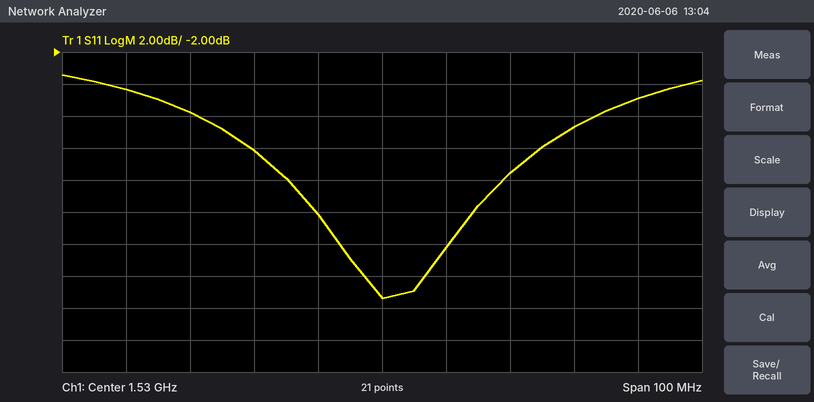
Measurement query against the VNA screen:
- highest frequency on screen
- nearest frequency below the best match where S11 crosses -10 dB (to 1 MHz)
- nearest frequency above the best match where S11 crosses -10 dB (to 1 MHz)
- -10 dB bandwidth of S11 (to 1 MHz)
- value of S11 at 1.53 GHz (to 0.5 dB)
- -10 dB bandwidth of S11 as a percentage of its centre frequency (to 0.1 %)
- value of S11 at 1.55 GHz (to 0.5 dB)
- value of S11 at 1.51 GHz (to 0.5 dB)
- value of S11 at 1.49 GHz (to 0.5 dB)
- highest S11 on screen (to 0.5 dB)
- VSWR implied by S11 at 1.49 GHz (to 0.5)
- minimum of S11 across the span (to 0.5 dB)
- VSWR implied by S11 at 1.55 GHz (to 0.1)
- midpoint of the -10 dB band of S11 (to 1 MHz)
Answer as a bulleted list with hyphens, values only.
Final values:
- 1.58 GHz
- 1.515 GHz
- 1.549 GHz
- 34 MHz
- -17.5 dB
- 2.2 %
- -9.5 dB
- -8.0 dB
- -4.5 dB
- -3.5 dB
- 4.0
- -17.5 dB
- 2.0
- 1.532 GHz
